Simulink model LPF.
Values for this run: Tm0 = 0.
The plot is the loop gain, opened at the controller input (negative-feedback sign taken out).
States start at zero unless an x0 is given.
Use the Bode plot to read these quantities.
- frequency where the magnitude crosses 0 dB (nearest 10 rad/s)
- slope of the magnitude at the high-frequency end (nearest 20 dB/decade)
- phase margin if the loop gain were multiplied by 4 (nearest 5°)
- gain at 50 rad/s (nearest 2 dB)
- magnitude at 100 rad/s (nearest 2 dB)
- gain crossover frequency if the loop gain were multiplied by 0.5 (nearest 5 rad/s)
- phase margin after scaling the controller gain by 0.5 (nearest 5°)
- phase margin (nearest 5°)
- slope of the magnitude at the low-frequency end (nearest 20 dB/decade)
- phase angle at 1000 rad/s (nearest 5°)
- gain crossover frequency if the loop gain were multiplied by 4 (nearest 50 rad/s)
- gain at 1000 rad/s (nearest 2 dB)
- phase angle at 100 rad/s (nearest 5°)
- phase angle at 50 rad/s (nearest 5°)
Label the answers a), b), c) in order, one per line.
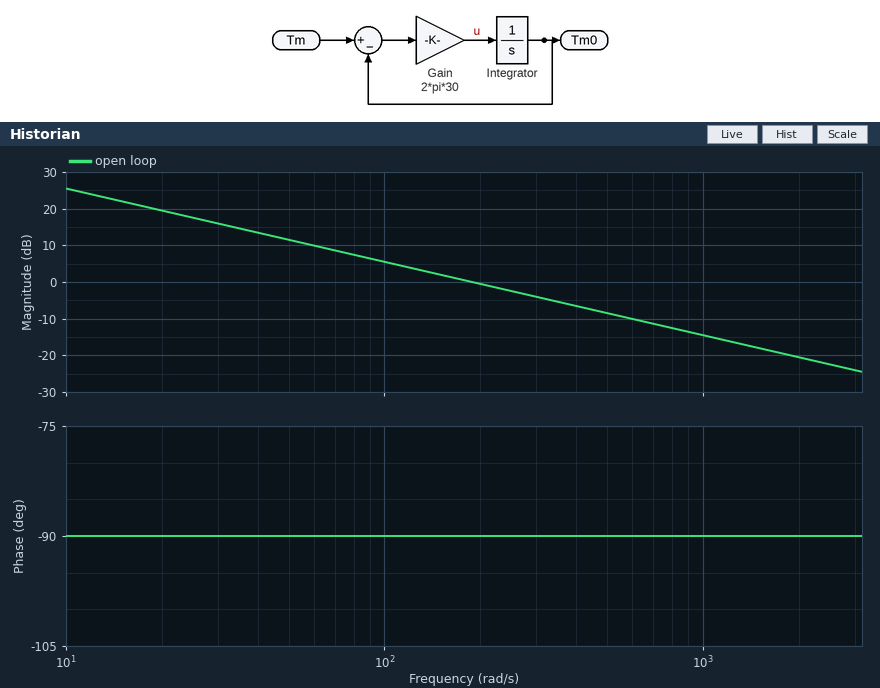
a) 190 rad/s
b) -20 dB/decade
c) 90°
d) 12 dB
e) 6 dB
f) 95 rad/s
g) 90°
h) 90°
i) -20 dB/decade
j) -90°
k) 750 rad/s
l) -14 dB
m) -90°
n) -90°
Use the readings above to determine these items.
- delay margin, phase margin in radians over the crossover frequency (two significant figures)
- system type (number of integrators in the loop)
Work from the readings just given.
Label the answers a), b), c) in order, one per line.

a) 0.0083 s
b) 1
